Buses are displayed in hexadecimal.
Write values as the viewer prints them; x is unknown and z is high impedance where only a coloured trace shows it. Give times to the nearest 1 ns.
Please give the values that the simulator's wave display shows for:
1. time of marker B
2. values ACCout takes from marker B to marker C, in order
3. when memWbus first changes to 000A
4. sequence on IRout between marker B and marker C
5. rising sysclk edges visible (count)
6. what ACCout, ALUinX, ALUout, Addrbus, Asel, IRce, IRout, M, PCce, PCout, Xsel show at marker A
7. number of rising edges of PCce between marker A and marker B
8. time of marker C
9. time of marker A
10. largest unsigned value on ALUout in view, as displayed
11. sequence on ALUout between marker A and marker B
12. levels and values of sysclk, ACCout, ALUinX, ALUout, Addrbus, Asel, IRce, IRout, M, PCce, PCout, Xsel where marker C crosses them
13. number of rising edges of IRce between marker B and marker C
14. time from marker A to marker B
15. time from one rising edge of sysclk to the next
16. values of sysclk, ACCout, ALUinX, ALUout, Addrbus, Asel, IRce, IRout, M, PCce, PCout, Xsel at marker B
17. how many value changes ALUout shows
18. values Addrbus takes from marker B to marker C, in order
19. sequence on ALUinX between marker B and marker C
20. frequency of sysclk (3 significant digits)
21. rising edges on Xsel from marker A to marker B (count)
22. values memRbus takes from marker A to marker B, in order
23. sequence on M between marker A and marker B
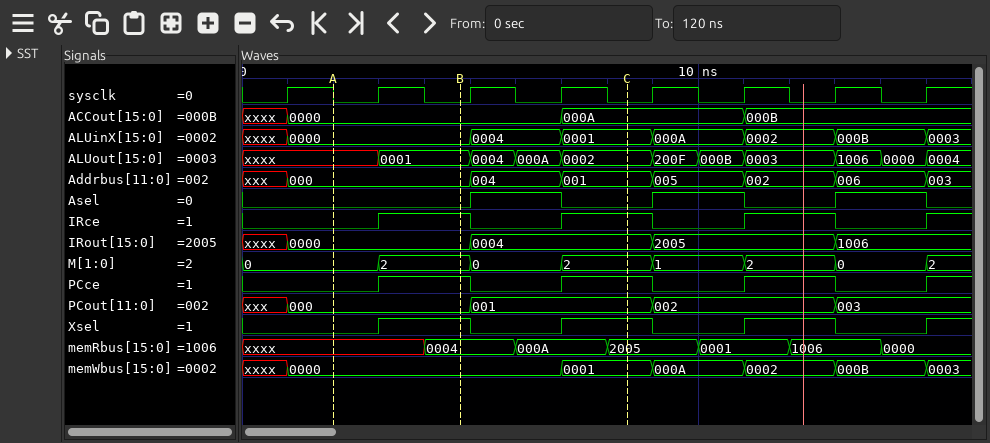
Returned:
5 ns
0000, 000A
9 ns
0000, 0004
8
ACCout=0000, ALUinX=0000, ALUout=xxxx, Addrbus=000, Asel=0, IRce=0, IRout=0000, M=0, PCce=0, PCout=000, Xsel=0
1
8 ns
2 ns
200F
xxxx, 0001
sysclk=0, ACCout=000A, ALUinX=0001, ALUout=0002, Addrbus=001, Asel=0, IRce=1, IRout=0004, M=2, PCce=1, PCout=001, Xsel=1
1
3 ns
2 ns
sysclk=0, ACCout=0000, ALUinX=0000, ALUout=0001, Addrbus=000, Asel=0, IRce=1, IRout=0000, M=2, PCce=1, PCout=000, Xsel=1
10
000, 004, 001
0000, 0004, 0001
500 MHz
1
xxxx, 0004
0, 2
